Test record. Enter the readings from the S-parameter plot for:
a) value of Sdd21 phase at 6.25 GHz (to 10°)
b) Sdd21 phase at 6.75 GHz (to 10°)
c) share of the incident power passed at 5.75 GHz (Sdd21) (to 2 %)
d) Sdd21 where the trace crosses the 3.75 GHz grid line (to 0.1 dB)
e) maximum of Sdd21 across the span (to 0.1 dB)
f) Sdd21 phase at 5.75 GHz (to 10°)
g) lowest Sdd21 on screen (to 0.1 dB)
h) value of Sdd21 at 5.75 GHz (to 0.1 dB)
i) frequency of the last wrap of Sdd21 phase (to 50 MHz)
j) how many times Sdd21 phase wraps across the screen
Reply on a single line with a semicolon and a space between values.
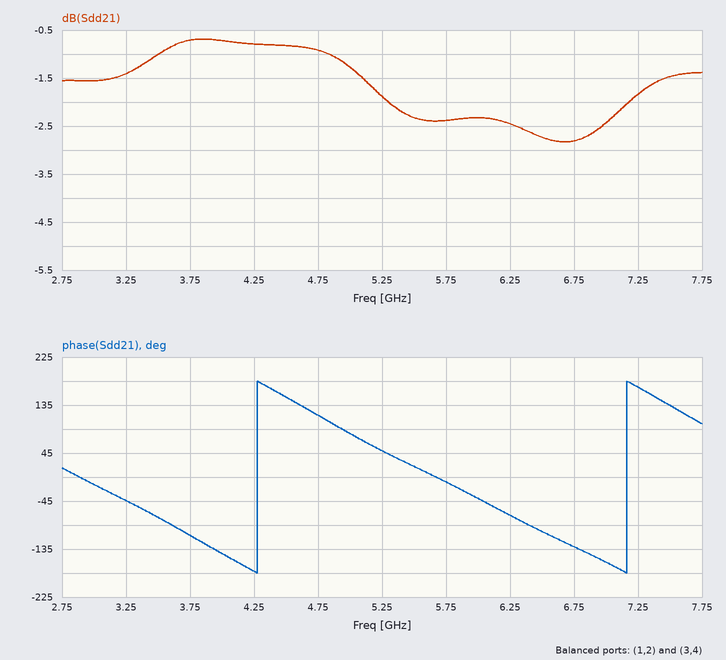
-70°; -130°; 58 %; -0.7 dB; -0.7 dB; -10°; -2.8 dB; -2.4 dB; 7.15 GHz; 2
